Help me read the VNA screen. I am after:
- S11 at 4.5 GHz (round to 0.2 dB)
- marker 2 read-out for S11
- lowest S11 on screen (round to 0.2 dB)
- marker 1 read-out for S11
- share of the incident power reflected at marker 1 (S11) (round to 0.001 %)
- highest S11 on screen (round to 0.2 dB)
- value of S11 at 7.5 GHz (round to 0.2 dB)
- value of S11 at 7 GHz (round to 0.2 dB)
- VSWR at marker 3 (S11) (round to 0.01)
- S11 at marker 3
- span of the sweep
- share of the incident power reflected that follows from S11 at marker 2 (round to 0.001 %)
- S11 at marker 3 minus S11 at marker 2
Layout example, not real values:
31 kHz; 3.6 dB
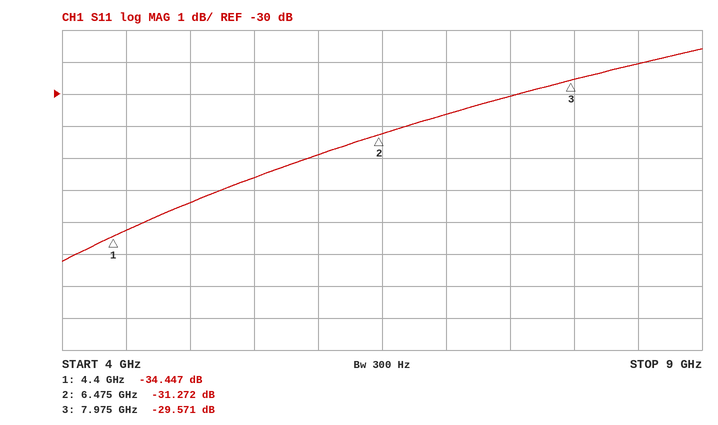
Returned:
-34.2 dB; -31.272 dB; -35.2 dB; -34.447 dB; 0.036 %; -28.6 dB; -30.0 dB; -30.6 dB; 1.07; -29.571 dB; 5 GHz; 0.075 %; 1.701 dB
